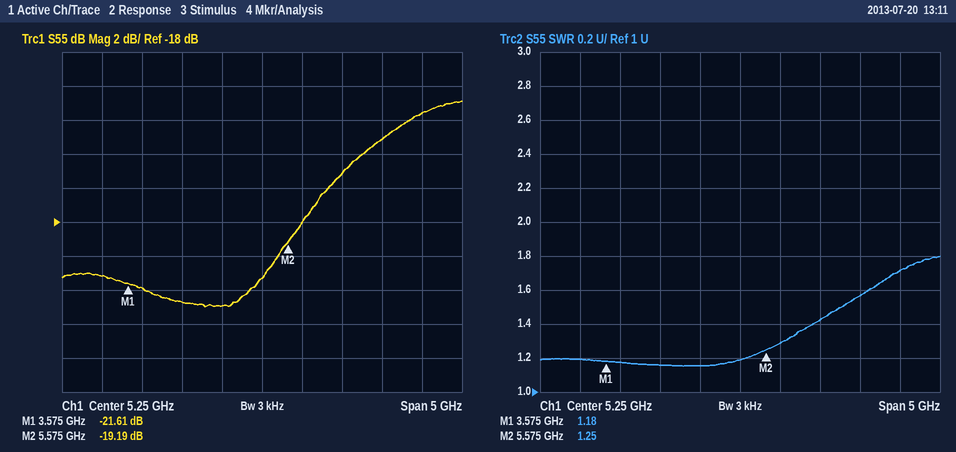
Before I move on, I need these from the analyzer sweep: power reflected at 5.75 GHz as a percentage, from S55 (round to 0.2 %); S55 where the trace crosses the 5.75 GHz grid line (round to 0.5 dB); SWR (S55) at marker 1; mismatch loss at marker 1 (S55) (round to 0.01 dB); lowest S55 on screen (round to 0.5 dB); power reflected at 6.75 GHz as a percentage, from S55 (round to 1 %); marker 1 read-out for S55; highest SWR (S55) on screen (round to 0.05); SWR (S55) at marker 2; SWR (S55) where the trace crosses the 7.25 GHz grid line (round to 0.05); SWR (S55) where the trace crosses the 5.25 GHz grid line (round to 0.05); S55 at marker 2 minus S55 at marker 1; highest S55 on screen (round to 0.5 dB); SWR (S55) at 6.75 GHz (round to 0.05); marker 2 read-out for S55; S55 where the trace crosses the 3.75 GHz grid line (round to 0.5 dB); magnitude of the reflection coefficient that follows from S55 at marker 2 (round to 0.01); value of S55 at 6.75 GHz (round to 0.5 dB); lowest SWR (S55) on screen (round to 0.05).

1.6 %
-18.0 dB
1.18
0.03 dB
-23.0 dB
5 %
-21.61 dB
1.80
1.25
1.70
1.20
2.42 dB
-11.0 dB
1.55
-19.19 dB
-22.0 dB
0.11
-13.0 dB
1.15
